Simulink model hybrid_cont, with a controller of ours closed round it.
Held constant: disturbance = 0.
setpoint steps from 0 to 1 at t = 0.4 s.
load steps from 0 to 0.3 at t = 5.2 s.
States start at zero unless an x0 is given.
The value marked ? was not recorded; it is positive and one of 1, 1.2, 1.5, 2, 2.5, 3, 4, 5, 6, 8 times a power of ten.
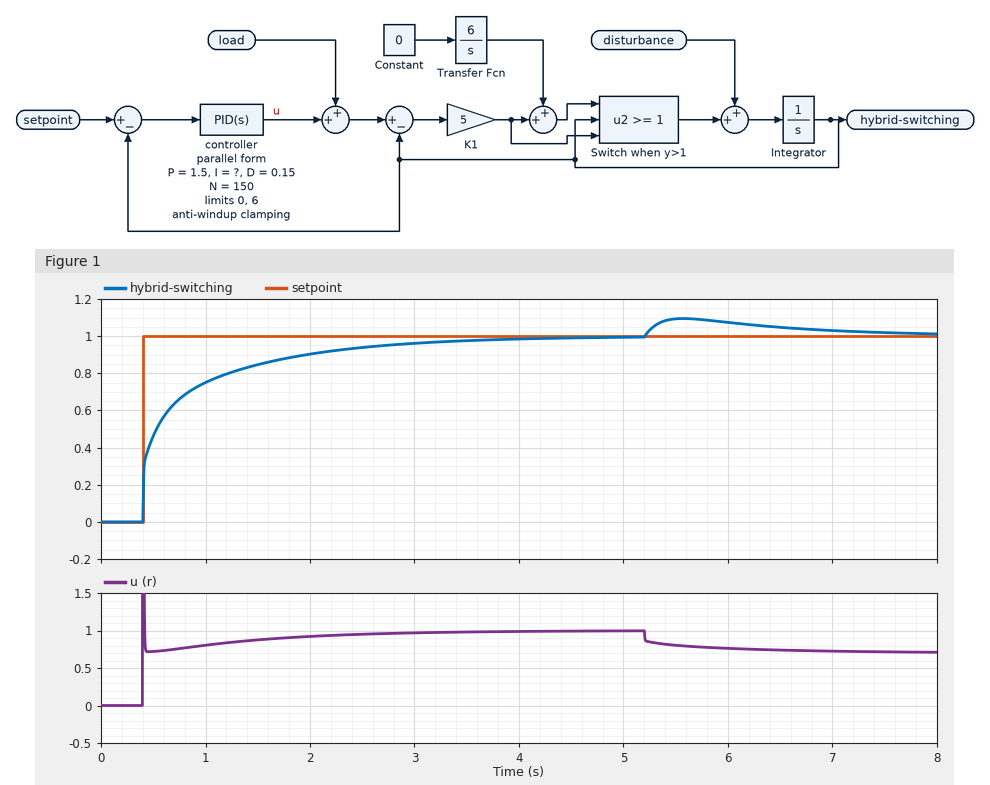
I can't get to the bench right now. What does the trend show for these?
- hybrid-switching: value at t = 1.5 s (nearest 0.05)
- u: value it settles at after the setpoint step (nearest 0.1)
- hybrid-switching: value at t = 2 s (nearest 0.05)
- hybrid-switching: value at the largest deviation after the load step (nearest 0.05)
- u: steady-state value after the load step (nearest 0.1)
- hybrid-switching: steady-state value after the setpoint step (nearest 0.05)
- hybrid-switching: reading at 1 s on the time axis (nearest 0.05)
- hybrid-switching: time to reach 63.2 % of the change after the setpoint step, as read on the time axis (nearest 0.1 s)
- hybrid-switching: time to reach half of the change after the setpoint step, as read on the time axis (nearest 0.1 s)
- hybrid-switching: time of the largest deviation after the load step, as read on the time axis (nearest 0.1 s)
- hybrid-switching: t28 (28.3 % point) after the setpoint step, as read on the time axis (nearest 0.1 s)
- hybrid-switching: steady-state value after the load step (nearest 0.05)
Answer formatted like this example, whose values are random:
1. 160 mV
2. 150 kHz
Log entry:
1. 0.85
2. 1.0
3. 0.90
4. 1.10
5. 0.7
6. 1.00
7. 0.75
8. 0.7 s
9. 0.5 s
10. 5.6 s
11. 0.4 s
12. 1.00
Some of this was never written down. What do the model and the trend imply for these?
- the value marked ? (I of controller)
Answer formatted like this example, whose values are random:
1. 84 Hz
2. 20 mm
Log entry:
1. 2
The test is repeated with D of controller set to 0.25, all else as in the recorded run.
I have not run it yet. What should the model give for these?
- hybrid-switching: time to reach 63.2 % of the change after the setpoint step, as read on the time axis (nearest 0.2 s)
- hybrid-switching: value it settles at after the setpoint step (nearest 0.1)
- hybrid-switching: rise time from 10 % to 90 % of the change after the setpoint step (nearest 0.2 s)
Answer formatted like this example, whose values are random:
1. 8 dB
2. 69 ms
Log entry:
1. 0.8 s
2. 1.0
3. 1.6 s
